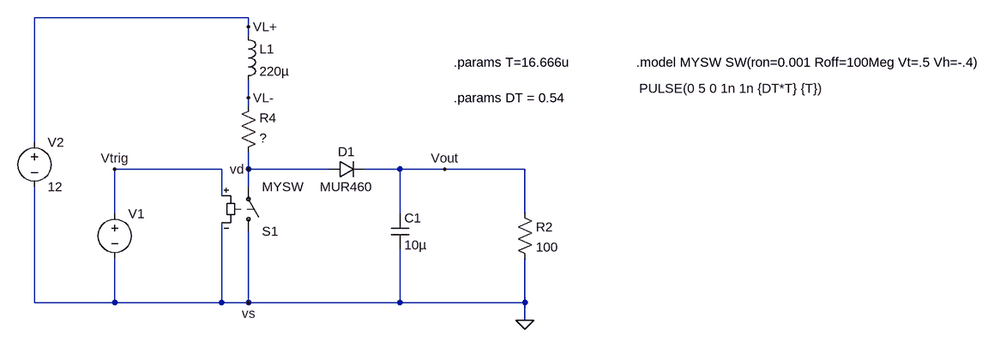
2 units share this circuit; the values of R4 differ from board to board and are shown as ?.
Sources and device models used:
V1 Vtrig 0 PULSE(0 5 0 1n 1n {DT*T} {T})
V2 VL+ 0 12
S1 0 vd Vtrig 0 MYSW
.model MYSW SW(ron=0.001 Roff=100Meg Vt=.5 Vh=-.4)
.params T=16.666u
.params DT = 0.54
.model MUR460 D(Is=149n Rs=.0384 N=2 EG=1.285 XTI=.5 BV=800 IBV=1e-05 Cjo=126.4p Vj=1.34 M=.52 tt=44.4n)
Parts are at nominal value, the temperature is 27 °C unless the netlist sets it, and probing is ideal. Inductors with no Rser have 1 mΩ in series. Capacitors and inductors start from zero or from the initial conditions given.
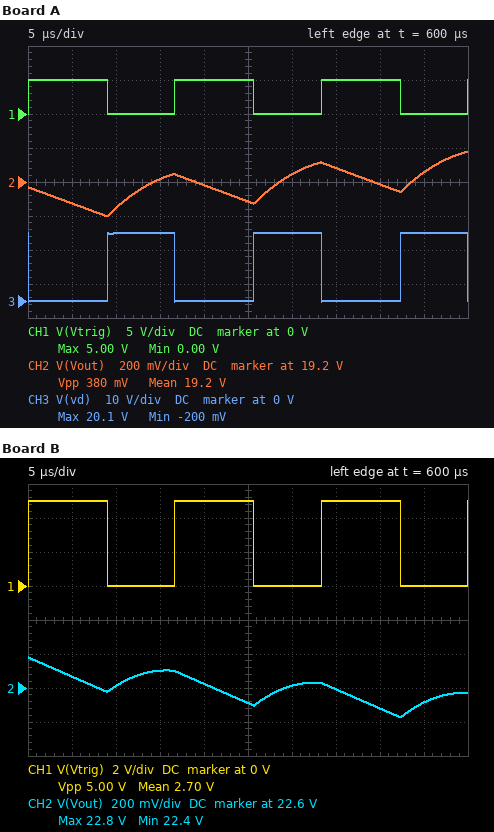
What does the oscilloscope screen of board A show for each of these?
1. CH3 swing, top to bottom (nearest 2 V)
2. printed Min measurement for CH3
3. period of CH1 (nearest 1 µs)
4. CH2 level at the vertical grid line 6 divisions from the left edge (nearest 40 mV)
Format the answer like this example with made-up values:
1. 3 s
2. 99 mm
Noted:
1. 20 V
2. -200 mV
3. 17 µs
4. 19.24 V
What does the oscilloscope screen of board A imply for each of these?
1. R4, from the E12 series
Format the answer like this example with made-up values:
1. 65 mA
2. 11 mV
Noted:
1. 5.6 Ω
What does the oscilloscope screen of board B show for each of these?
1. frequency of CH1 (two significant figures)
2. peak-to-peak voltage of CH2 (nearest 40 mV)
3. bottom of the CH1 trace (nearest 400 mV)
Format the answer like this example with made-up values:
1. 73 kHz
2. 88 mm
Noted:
1. 60 kHz
2. 360 mV
3. 0 V
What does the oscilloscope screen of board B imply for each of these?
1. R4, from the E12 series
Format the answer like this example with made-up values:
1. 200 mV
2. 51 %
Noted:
1. 2.7 Ω
